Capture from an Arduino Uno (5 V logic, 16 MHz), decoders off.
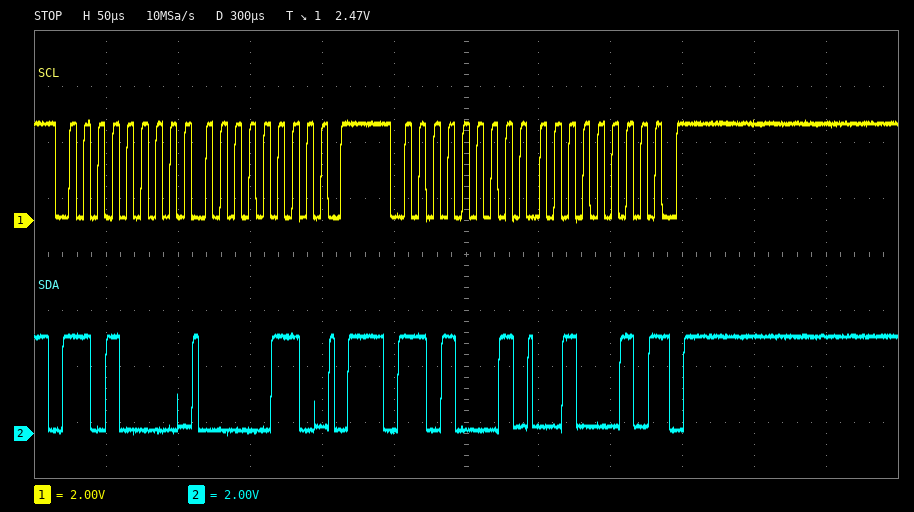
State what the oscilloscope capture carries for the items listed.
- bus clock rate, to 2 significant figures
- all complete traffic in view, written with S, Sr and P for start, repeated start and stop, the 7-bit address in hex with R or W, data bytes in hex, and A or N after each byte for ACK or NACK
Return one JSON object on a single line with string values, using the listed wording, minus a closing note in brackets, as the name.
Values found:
{"bus clock rate, to 2 significant figures": "100 kHz", "all complete traffic in view, written with S, Sr and P for start, repeated start and stop, the 7-bit address in hex with R or W, data bytes in hex, and A or N after each byte for ACK or NACK": "S 68W A 06 A P S 68R A 22 N P"}
